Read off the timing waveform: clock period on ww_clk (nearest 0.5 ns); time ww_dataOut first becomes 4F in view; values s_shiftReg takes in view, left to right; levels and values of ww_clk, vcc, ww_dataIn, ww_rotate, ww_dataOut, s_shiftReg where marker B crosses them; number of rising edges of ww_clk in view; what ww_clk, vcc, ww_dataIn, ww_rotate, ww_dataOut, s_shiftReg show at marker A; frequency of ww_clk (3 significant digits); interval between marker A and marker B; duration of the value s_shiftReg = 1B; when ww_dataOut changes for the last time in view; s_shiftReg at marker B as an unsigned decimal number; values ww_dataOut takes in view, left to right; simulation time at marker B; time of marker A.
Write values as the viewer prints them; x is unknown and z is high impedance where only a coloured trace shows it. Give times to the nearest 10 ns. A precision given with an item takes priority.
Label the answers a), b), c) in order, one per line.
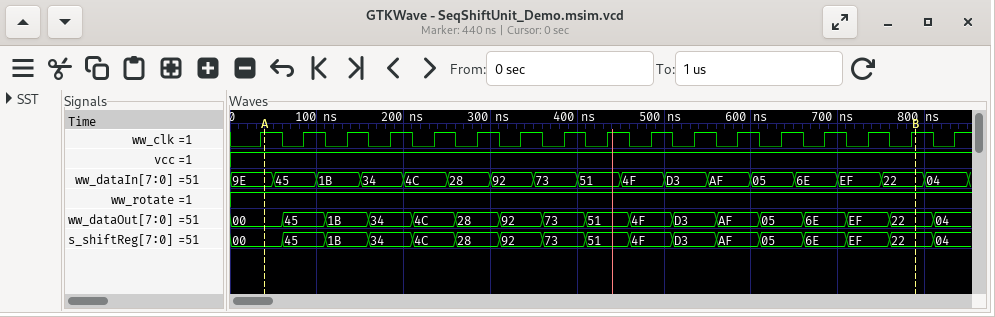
a) 50 ns
b) 460 ns
c) 00, 45, 1B, 34, 4C, 28, 92, 73, 51, 4F, D3, AF, 05, 6E, EF, 22, 04
d) ww_clk=1, vcc=1, ww_dataIn=22, ww_rotate=1, ww_dataOut=22, s_shiftReg=22
e) 17
f) ww_clk=1, vcc=1, ww_dataIn=9E, ww_rotate=1, ww_dataOut=00, s_shiftReg=00
g) 20.0 MHz
h) 750 ns
i) 50 ns
j) 810 ns
k) 34
l) 00, 45, 1B, 34, 4C, 28, 92, 73, 51, 4F, D3, AF, 05, 6E, EF, 22, 04
m) 790 ns
n) 40 ns
